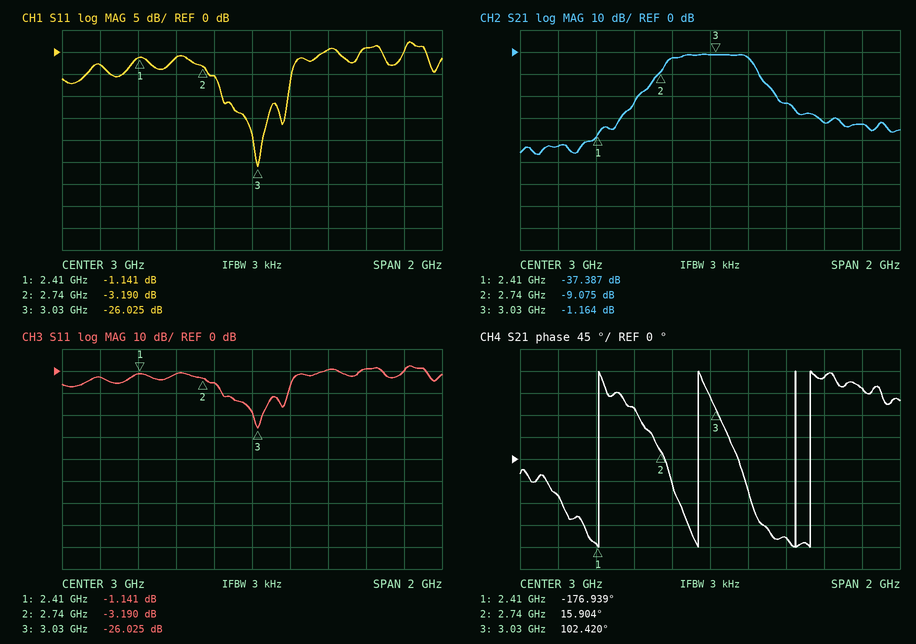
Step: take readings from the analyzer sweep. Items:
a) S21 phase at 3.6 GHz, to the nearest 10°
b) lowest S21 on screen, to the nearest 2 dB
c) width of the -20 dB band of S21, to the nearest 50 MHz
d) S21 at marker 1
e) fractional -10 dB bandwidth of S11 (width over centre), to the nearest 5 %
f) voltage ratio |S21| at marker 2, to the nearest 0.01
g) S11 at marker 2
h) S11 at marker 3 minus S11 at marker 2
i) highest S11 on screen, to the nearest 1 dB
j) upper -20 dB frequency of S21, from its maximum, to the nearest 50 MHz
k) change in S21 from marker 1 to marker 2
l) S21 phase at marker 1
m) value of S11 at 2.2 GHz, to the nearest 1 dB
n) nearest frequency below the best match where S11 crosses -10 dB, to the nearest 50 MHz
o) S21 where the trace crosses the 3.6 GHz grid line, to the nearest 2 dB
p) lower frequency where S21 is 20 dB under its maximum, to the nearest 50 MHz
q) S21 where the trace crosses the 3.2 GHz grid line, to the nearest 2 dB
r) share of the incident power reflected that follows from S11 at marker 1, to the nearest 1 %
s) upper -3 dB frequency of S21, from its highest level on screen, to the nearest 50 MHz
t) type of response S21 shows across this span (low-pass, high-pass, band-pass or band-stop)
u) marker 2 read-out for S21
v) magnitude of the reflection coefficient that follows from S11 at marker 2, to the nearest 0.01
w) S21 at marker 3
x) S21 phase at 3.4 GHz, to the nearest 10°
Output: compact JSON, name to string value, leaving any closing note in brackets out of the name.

{"S21 phase at 3.6 GHz, to the nearest 10°": "170°", "lowest S21 on screen, to the nearest 2 dB": "-46 dB", "width of the -20 dB band of S21, to the nearest 50 MHz": "750 MHz", "S21 at marker 1": "-37.387 dB", "fractional -10 dB bandwidth of S11 (width over centre), to the nearest 5 %": "10 %", "voltage ratio |S21| at marker 2, to the nearest 0.01": "0.35", "S11 at marker 2": "-3.190 dB", "S11 at marker 3 minus S11 at marker 2": "-22.835 dB", "highest S11 on screen, to the nearest 1 dB": "2 dB", "upper -20 dB frequency of S21, from its maximum, to the nearest 50 MHz": "3.35 GHz", "change in S21 from marker 1 to marker 2": "28.312 dB", "S21 phase at marker 1": "-176.939°", "value of S11 at 2.2 GHz, to the nearest 1 dB": "-3 dB", "nearest frequency below the best match where S11 crosses -10 dB, to the nearest 50 MHz": "2.85 GHz", "S21 where the trace crosses the 3.6 GHz grid line, to the nearest 2 dB": "-32 dB", "lower frequency where S21 is 20 dB under its maximum, to the nearest 50 MHz": "2.60 GHz", "S21 where the trace crosses the 3.2 GHz grid line, to the nearest 2 dB": "-2 dB", "share of the incident power reflected that follows from S11 at marker 1, to the nearest 1 %": "77 %", "upper -3 dB frequency of S21, from its highest level on screen, to the nearest 50 MHz": "3.20 GHz", "type of response S21 shows across this span": "band-pass", "marker 2 read-out for S21": "-9.075 dB", "magnitude of the reflection coefficient that follows from S11 at marker 2, to the nearest 0.01": "0.69", "S21 at marker 3": "-1.164 dB", "S21 phase at 3.4 GHz, to the nearest 10°": "-160°"}
